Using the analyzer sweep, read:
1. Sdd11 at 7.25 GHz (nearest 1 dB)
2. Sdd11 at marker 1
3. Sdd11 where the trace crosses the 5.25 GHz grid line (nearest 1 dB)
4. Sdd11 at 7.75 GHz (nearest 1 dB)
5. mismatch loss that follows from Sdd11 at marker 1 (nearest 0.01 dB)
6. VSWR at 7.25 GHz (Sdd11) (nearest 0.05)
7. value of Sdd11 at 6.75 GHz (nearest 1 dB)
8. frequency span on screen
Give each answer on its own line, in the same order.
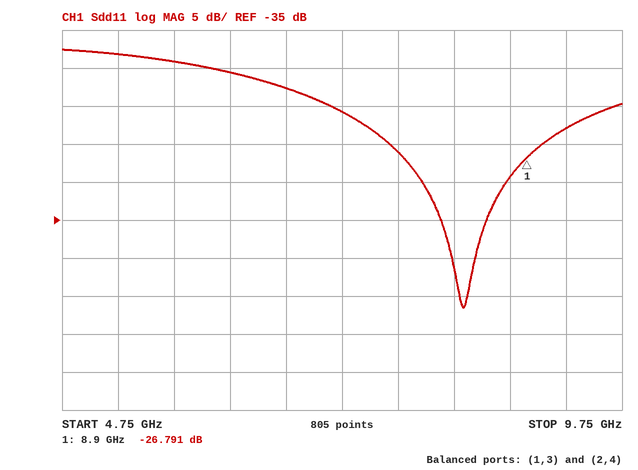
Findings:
-21 dB
-26.791 dB
-13 dB
-26 dB
0.01 dB
1.20
-18 dB
5 GHz
